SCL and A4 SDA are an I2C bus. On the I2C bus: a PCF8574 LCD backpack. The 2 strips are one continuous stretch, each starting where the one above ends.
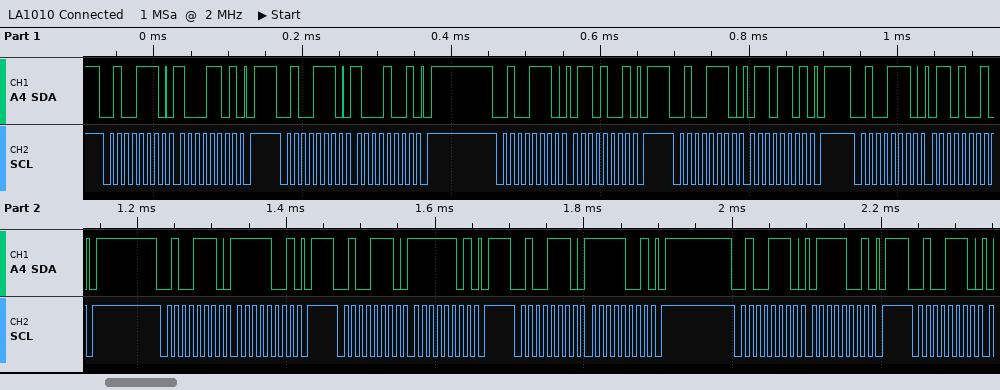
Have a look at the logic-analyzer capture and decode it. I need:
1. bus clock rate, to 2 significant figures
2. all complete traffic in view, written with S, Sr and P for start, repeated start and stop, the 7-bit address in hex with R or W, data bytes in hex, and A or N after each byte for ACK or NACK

100 kHz
S 27W A 8D A P S 27W A 89 A P S 27W A 69 A P S 27W A 6D A P S 27W A 69 A P S 27W A F9 A P S 27W A FD A P S 27W A F9 A P S 27W A 79 A P S 27W A
